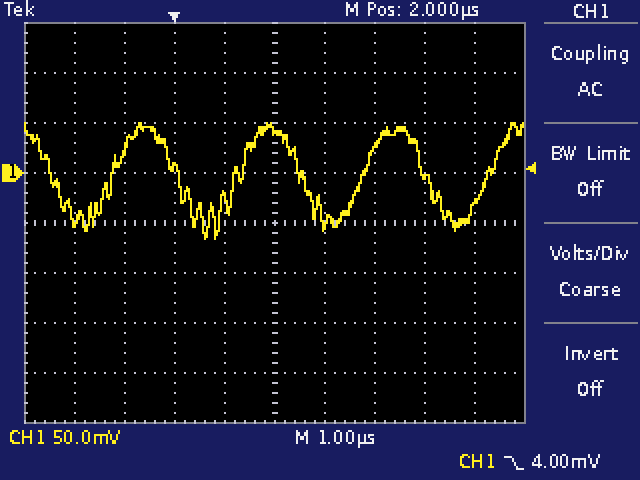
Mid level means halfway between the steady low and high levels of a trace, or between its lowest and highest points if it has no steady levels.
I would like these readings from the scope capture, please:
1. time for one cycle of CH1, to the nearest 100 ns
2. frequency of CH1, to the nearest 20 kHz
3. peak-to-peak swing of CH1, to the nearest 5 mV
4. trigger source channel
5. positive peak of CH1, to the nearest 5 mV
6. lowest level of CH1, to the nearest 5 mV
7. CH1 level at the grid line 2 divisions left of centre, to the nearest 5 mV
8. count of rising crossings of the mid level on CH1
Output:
2.5 µs
400 kHz
115 mV
CH1
50 mV
-65 mV
5 mV
4
